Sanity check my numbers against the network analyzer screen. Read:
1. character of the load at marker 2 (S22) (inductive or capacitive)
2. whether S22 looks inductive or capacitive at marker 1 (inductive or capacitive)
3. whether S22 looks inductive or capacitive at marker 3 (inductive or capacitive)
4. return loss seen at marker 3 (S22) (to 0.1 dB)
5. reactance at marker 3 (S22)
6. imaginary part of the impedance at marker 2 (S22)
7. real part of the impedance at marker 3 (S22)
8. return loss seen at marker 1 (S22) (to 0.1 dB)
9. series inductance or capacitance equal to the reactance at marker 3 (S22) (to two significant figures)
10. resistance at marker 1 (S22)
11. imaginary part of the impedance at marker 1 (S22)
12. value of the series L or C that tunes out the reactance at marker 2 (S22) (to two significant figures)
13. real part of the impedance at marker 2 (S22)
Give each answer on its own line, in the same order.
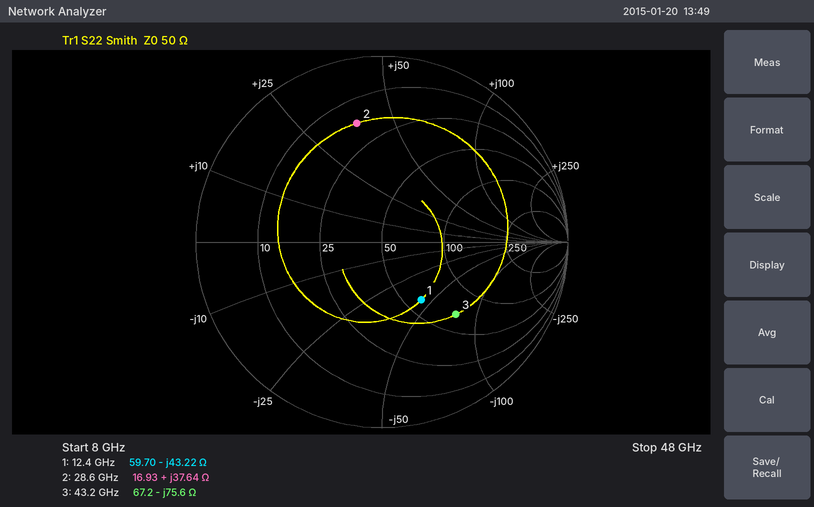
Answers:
inductive
capacitive
capacitive
5.1 dB
-75.6 Ω
+37.64 Ω
67.2 Ω
8.5 dB
49 fF
59.70 Ω
-43.22 Ω
150 fF
16.93 Ω
